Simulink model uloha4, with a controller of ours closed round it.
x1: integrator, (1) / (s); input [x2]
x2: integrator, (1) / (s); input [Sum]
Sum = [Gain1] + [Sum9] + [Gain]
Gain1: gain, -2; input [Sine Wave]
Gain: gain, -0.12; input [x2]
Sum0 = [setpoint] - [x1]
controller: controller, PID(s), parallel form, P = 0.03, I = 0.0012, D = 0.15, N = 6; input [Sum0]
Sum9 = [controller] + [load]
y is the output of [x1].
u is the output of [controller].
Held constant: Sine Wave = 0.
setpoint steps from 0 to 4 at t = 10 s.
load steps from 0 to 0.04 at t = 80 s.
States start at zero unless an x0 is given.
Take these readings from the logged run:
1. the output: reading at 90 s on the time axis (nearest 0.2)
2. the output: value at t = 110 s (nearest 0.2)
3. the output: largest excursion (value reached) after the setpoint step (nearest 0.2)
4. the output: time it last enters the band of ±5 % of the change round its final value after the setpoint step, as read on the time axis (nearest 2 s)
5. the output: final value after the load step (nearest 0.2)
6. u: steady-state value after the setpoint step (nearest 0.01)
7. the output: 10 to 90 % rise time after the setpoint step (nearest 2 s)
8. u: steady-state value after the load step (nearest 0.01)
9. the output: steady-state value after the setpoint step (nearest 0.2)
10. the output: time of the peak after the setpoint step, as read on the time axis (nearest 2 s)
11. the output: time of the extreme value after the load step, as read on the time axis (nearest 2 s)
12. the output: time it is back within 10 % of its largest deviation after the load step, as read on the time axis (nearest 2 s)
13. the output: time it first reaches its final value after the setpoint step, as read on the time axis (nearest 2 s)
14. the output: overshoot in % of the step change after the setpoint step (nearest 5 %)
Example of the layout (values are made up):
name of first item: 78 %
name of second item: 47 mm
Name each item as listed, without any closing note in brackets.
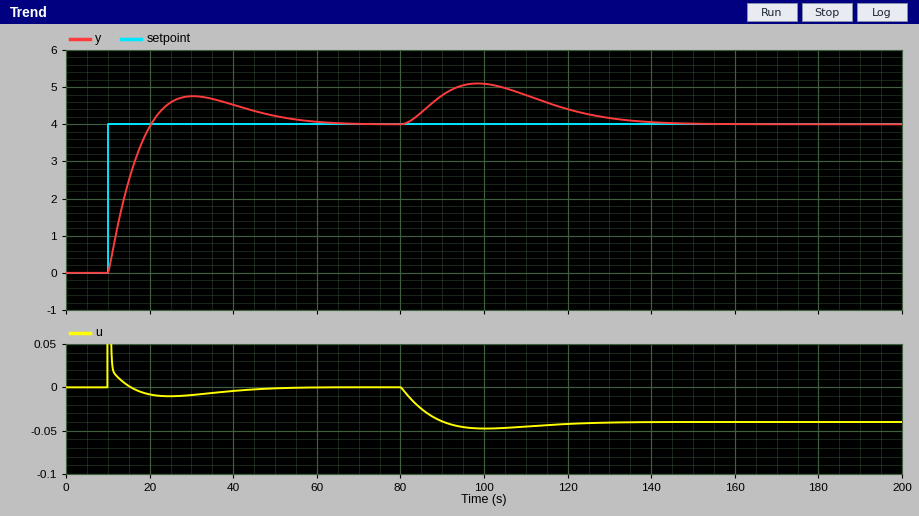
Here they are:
the output: reading at 90 s on the time axis: 4.8
the output: value at t = 110 s: 4.8
the output: largest excursion (value reached) after the setpoint step: 4.8
the output: time it last enters the band of ±5 % of the change round its final value after the setpoint step, as read on the time axis: 52 s
the output: final value after the load step: 4.0
u: steady-state value after the setpoint step: 0.00
the output: 10 to 90 % rise time after the setpoint step: 8 s
u: steady-state value after the load step: -0.04
the output: steady-state value after the setpoint step: 4.0
the output: time of the peak after the setpoint step, as read on the time axis: 30 s
the output: time of the extreme value after the load step, as read on the time axis: 98 s
the output: time it is back within 10 % of its largest deviation after the load step, as read on the time axis: 134 s
the output: time it first reaches its final value after the setpoint step, as read on the time axis: 20 s
the output: overshoot in % of the step change after the setpoint step: 20 %
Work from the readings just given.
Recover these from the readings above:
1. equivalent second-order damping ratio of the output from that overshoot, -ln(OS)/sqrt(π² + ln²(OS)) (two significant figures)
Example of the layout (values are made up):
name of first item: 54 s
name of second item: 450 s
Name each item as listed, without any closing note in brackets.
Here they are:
equivalent second-order damping ratio of the output from that overshoot, -ln(OS)/sqrt(π² + ln²(OS)): 0.46
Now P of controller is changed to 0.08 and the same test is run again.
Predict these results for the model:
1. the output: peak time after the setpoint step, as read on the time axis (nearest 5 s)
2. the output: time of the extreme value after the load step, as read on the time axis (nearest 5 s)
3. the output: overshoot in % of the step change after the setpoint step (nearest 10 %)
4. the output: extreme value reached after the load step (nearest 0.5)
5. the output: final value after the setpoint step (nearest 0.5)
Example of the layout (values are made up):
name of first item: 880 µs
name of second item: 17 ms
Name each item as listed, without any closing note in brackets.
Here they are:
the output: peak time after the setpoint step, as read on the time axis: 20 s
the output: time of the extreme value after the load step, as read on the time axis: 90 s
the output: overshoot in % of the step change after the setpoint step: 30 %
the output: extreme value reached after the load step: 4.5
the output: final value after the setpoint step: 4.0
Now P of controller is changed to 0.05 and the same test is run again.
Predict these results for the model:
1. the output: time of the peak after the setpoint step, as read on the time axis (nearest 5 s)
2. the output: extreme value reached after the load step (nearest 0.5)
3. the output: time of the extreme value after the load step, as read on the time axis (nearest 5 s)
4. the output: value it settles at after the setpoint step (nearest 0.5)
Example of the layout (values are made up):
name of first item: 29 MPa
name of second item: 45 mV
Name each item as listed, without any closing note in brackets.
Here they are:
the output: time of the peak after the setpoint step, as read on the time axis: 25 s
the output: extreme value reached after the load step: 5.0
the output: time of the extreme value after the load step, as read on the time axis: 95 s
the output: value it settles at after the setpoint step: 4.0
